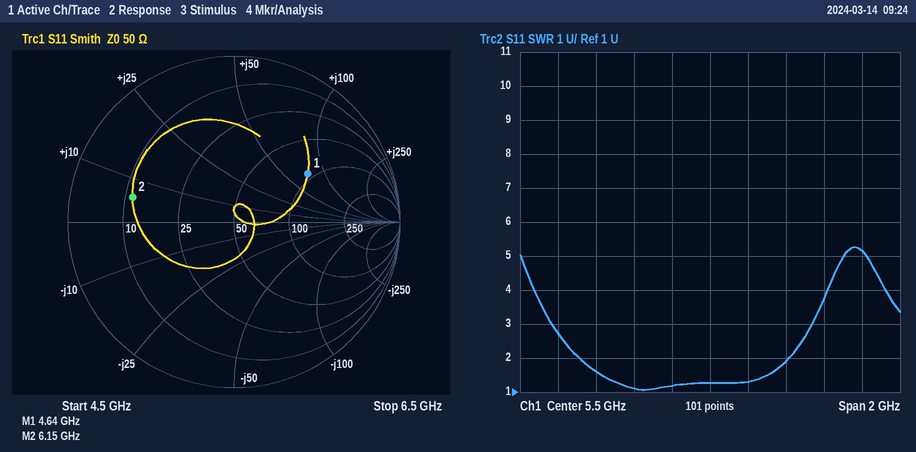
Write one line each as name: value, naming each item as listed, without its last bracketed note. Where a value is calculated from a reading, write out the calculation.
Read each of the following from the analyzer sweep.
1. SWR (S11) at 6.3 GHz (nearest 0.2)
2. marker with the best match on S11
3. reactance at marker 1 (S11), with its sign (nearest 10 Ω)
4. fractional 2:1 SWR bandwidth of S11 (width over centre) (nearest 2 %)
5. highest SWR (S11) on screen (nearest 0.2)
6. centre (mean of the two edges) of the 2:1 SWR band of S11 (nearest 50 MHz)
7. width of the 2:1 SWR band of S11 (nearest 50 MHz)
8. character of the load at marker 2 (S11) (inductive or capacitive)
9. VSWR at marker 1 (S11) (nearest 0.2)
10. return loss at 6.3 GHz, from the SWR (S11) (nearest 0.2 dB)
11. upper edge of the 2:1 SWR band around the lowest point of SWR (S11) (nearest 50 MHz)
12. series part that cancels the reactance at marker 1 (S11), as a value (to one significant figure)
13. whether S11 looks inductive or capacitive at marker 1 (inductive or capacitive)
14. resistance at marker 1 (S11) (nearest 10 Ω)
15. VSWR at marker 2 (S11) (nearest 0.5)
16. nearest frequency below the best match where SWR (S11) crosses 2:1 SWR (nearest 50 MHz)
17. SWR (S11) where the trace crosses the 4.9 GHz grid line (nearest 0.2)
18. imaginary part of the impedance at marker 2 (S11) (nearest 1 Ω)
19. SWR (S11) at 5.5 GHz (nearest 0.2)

SWR (S11) at 6.3 GHz: 5.2
marker with the best match on S11: marker 1
reactance at marker 1 (S11), with its sign: +70 Ω
fractional 2:1 SWR bandwidth of S11 (width over centre): 1.1 GHz / 5.35 GHz ≈ 20.6 %, so 20 % to the nearest 2 %
highest SWR (S11) on screen: 5.2
centre (mean of the two edges) of the 2:1 SWR band of S11: 5.35 GHz
width of the 2:1 SWR band of S11: 5.90 GHz − 4.80 GHz = 1.10 GHz
character of the load at marker 2 (S11): inductive
VSWR at marker 1 (S11): 3.2
return loss at 6.3 GHz, from the SWR (S11): −20 log10((5.2 − 1)/(5.2 + 1)) ≈ 3.4 dB
upper edge of the 2:1 SWR band around the lowest point of SWR (S11): 5.90 GHz
series part that cancels the reactance at marker 1 (S11), as a value: C = 1/(2π × 4.64 GHz × 70 Ω) ≈ 490 fF, so 500 fF to one significant figure
whether S11 looks inductive or capacitive at marker 1: inductive
resistance at marker 1 (S11): 90 Ω
VSWR at marker 2 (S11): 4.5
nearest frequency below the best match where SWR (S11) crosses 2:1 SWR: 4.80 GHz
SWR (S11) where the trace crosses the 4.9 GHz grid line: 1.6
imaginary part of the impedance at marker 2 (S11): +6 Ω
SWR (S11) at 5.5 GHz: 1.2
